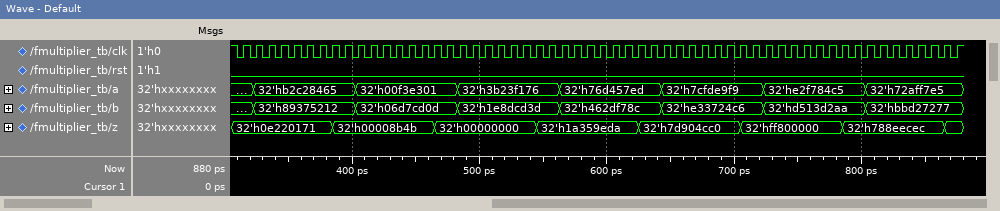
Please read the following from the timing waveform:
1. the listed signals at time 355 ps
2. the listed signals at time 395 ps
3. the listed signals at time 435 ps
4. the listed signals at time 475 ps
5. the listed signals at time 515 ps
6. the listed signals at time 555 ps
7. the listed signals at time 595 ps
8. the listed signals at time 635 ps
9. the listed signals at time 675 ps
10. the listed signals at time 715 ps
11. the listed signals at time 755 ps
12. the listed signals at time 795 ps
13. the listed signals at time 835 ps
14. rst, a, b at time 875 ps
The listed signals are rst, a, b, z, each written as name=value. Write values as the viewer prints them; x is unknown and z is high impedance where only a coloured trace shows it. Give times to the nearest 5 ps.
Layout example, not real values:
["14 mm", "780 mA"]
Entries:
["rst=0, a=32'hb2c28465, b=32'h89375212, z=32'h0e220171", "rst=0, a=32'hb2c28465, b=32'h89375212, z=32'h00008b4b", "rst=0, a=32'h00f3e301, b=32'h06d7cd0d, z=32'h00008b4b", "rst=0, a=32'h00f3e301, b=32'h06d7cd0d, z=32'h00000000", "rst=0, a=32'h3b23f176, b=32'h1e8dcd3d, z=32'h00000000", "rst=0, a=32'h3b23f176, b=32'h1e8dcd3d, z=32'h1a359eda", "rst=0, a=32'h76d457ed, b=32'h462df78c, z=32'h1a359eda", "rst=0, a=32'h76d457ed, b=32'h462df78c, z=32'h7d904cc0", "rst=0, a=32'h7cfde9f9, b=32'he33724c6, z=32'h7d904cc0", "rst=0, a=32'h7cfde9f9, b=32'he33724c6, z=32'hff800000", "rst=0, a=32'he2f784c5, b=32'hd513d2aa, z=32'hff800000", "rst=0, a=32'he2f784c5, b=32'hd513d2aa, z=32'h788eecec", "rst=0, a=32'h72aff7e5, b=32'hbbd27277, z=32'h788eecec", "rst=0, a=32'h72aff7e5, b=32'hbbd27277"]
